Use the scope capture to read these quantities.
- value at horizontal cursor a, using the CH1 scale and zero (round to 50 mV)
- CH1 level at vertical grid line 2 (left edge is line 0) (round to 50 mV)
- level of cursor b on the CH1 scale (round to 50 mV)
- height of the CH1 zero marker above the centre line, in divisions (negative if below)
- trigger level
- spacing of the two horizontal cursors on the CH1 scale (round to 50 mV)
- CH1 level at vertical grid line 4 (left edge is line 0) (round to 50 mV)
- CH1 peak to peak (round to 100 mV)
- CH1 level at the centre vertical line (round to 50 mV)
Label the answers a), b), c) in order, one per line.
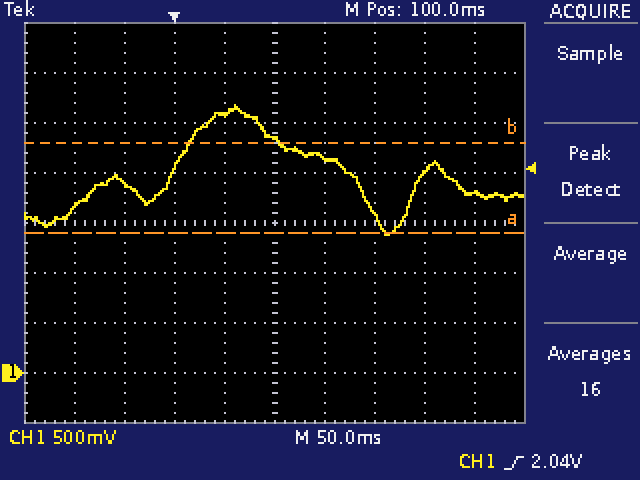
a) 1.40 V
b) 1.90 V
c) 2.30 V
d) -3.0 div
e) 2.04 V
f) 900 mV
g) 2.60 V
h) 1.30 V
i) 2.35 V
